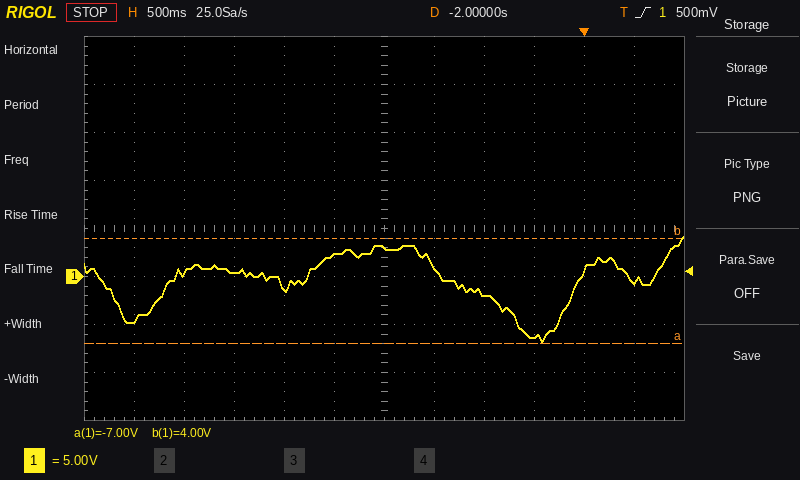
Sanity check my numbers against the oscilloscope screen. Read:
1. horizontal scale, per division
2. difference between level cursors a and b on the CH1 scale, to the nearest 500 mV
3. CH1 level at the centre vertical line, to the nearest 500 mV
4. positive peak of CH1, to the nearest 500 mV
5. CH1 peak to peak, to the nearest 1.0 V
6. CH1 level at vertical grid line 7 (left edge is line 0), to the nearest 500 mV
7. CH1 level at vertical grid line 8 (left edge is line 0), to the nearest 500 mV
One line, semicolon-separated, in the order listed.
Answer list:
500 ms; 11.0 V; 3.0 V; 4.0 V; 11.0 V; 1.0 V; -2.0 V
